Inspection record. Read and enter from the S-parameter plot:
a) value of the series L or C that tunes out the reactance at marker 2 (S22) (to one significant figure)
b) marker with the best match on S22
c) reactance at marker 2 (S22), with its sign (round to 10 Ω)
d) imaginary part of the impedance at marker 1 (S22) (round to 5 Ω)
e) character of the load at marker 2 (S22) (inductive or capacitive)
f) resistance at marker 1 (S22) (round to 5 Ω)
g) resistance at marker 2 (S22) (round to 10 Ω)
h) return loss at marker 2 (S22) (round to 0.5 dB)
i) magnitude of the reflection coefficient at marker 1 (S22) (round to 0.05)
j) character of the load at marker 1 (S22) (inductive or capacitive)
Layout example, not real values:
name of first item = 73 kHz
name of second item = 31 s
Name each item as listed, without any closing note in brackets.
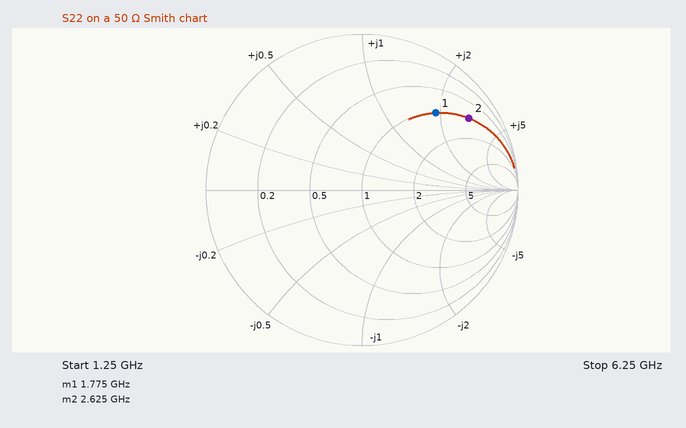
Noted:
value of the series L or C that tunes out the reactance at marker 2 (S22) = 400 fF
marker with the best match on S22 = marker 1
reactance at marker 2 (S22), with its sign = +150 Ω
imaginary part of the impedance at marker 1 (S22) = +95 Ω
character of the load at marker 2 (S22) = inductive
resistance at marker 1 (S22) = 50 Ω
resistance at marker 2 (S22) = 50 Ω
return loss at marker 2 (S22) = 1.5 dB
magnitude of the reflection coefficient at marker 1 (S22) = 0.70
character of the load at marker 1 (S22) = inductive
